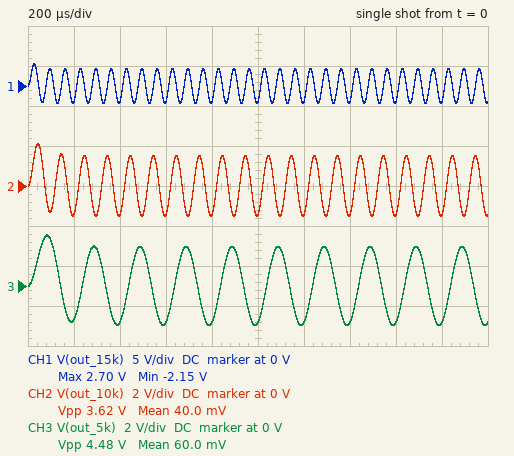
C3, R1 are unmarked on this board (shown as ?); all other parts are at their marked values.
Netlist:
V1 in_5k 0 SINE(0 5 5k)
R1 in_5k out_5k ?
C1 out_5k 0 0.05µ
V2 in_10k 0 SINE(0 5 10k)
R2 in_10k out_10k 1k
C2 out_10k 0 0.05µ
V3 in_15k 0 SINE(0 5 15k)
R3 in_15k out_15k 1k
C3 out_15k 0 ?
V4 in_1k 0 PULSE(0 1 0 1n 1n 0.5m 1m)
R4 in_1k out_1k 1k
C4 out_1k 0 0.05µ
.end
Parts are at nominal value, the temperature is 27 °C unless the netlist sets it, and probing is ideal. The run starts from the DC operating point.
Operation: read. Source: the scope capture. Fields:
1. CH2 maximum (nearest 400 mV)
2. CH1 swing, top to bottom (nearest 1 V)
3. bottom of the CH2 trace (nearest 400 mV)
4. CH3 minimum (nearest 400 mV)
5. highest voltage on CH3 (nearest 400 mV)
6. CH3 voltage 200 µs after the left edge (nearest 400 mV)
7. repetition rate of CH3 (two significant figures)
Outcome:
2.0 V
5 V
-1.6 V
-2.0 V
2.4 V
-1.6 V
5.0 kHz
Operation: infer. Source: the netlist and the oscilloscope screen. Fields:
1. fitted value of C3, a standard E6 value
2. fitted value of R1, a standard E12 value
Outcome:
22 nF
1.5 kΩ
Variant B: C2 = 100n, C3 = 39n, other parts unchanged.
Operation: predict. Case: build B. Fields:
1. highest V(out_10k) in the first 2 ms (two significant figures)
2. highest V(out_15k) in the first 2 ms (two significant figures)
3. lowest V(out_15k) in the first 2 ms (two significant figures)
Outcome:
1.3 V
1.9 V
-1.3 V
